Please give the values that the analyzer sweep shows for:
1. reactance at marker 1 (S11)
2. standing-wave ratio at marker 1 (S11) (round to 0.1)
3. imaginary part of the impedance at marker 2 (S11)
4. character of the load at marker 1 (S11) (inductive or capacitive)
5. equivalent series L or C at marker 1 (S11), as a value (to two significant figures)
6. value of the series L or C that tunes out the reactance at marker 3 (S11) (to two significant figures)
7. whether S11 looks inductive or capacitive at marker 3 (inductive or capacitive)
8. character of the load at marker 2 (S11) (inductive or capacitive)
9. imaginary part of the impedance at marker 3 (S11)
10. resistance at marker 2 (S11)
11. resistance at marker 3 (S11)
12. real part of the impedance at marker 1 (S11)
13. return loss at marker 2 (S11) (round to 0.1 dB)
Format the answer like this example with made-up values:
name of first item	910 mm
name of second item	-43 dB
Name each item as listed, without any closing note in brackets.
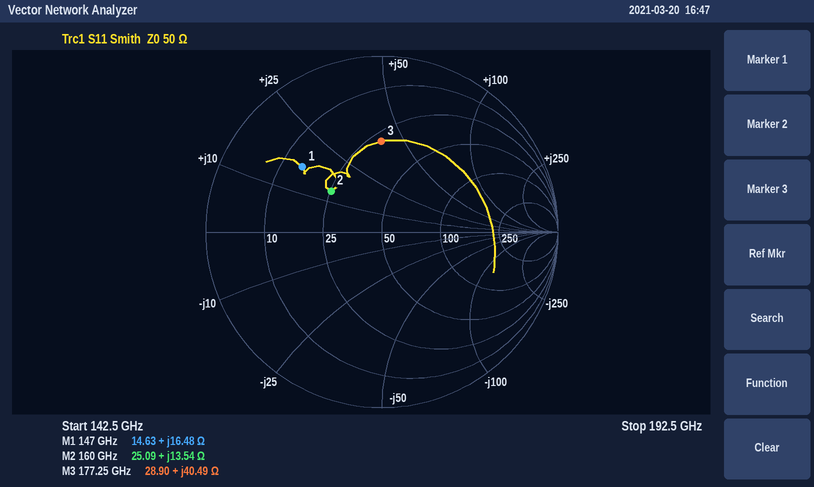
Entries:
reactance at marker 1	+16.48 Ω
standing-wave ratio at marker 1 (S11)	3.8
imaginary part of the impedance at marker 2	+13.54 Ω
character of the load at marker 1 (S11)	inductive
equivalent series L or C at marker 1 (S11), as a value	18 pH
value of the series L or C that tunes out the reactance at marker 3 (S11)	22 fF
whether S11 looks inductive or capacitive at marker 3	inductive
character of the load at marker 2 (S11)	inductive
imaginary part of the impedance at marker 3	+40.49 Ω
resistance at marker 2	25.09 Ω
resistance at marker 3	28.90 Ω
real part of the impedance at marker 1	14.63 Ω
return loss at marker 2 (S11)	8.6 dB
